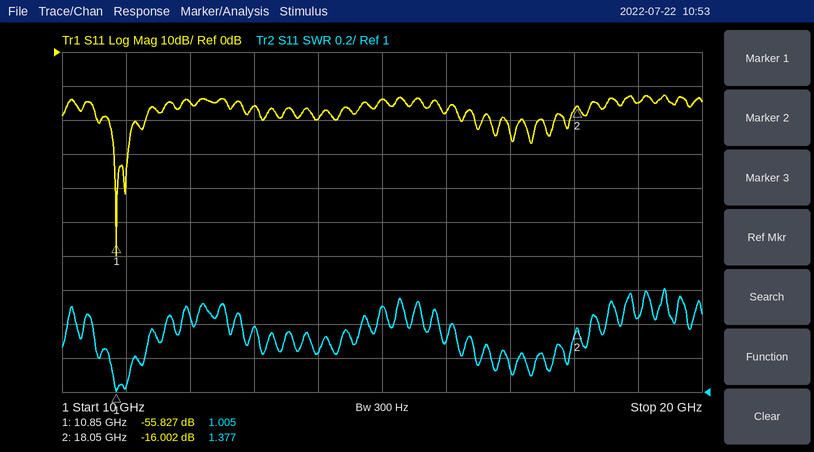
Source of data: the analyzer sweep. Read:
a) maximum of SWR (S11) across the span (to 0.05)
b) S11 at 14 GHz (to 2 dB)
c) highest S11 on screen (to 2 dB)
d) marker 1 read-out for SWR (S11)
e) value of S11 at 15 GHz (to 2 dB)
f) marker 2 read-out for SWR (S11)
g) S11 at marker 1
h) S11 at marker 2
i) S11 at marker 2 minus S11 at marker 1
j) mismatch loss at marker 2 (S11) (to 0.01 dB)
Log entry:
1.60
-20 dB
-12 dB
1.005
-14 dB
1.377
-55.827 dB
-16.002 dB
39.825 dB
0.11 dB
